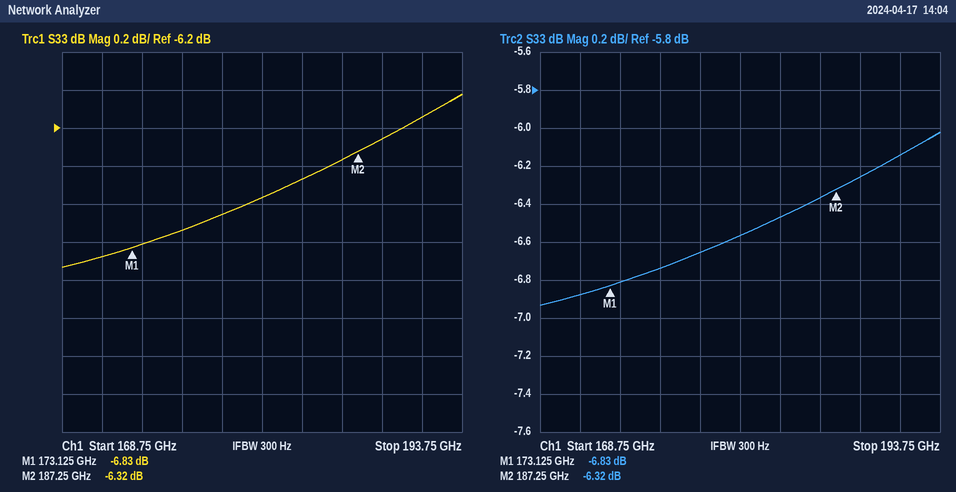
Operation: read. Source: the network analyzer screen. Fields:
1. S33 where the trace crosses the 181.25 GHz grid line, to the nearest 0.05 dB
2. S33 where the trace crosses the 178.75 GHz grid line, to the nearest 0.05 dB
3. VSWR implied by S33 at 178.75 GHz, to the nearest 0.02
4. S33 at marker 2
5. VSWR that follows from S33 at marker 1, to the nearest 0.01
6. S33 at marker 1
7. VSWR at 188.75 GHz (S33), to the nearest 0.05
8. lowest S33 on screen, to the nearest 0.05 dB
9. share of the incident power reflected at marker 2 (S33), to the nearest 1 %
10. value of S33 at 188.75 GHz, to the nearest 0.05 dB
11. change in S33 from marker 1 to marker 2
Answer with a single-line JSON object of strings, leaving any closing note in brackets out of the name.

{"S33 where the trace crosses the 181.25 GHz grid line, to the nearest 0.05 dB": "-6.55 dB", "S33 where the trace crosses the 178.75 GHz grid line, to the nearest 0.05 dB": "-6.65 dB", "VSWR implied by S33 at 178.75 GHz, to the nearest 0.02": "2.74", "S33 at marker 2": "-6.32 dB", "VSWR that follows from S33 at marker 1, to the nearest 0.01": "2.67", "S33 at marker 1": "-6.83 dB", "VSWR at 188.75 GHz (S33), to the nearest 0.05": "2.90", "lowest S33 on screen, to the nearest 0.05 dB": "-6.95 dB", "share of the incident power reflected at marker 2 (S33), to the nearest 1 %": "23 %", "value of S33 at 188.75 GHz, to the nearest 0.05 dB": "-6.25 dB", "change in S33 from marker 1 to marker 2": "0.51 dB"}
